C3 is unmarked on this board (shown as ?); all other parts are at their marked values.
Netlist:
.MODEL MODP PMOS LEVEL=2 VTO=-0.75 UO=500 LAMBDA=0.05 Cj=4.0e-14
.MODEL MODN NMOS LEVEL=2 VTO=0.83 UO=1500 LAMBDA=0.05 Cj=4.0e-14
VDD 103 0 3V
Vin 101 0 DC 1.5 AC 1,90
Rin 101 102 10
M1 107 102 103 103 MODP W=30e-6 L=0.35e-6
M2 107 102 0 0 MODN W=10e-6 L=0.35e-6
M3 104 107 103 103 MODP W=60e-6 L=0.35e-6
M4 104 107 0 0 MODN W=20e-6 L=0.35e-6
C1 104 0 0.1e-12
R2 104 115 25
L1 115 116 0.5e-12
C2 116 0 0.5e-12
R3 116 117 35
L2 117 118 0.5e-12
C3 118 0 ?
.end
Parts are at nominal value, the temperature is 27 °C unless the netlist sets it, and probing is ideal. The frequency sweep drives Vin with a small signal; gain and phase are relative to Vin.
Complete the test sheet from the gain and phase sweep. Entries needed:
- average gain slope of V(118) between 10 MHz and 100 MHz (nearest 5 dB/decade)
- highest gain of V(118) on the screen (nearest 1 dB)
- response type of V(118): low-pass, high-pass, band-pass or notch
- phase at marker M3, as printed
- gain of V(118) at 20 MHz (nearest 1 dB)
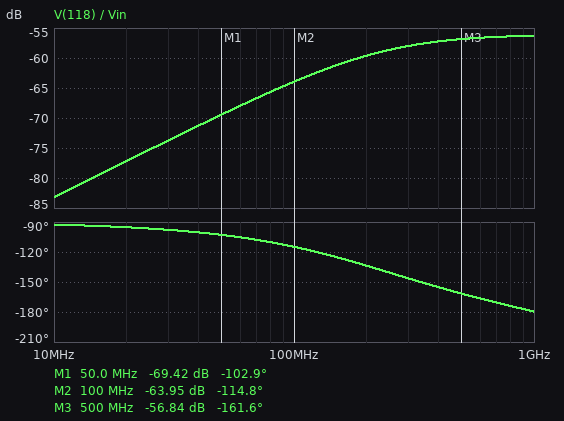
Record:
20 dB/decade
-56 dB
high-pass
-161.6 deg
-77 dB
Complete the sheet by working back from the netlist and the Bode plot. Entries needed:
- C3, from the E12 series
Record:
2.2 pF
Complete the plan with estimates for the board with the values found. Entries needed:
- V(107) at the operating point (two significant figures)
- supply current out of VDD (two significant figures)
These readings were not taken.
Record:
2.5 V
380 µA
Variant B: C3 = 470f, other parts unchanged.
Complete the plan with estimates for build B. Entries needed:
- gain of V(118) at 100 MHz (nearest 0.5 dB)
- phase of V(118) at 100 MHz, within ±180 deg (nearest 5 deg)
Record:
-63.5 dB
-100 deg
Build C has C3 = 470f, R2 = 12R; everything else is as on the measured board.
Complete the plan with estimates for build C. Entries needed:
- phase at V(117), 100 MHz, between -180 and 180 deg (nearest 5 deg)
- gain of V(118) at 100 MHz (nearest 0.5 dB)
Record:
-100 deg
-63.5 dB
